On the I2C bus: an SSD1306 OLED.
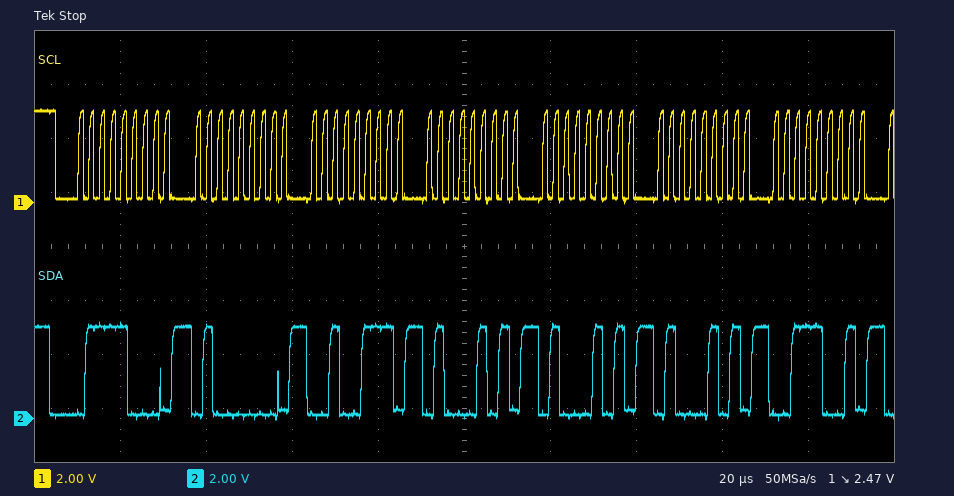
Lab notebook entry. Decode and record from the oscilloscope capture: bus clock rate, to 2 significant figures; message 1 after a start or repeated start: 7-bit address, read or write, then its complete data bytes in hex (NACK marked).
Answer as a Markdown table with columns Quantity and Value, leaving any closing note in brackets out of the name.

| Quantity | Value |
|---|---|
| bus clock rate, to 2 significant figures | 400 kHz |
| message 1 after a start or repeated start: 7-bit address, read or write, then its complete data bytes in hex | 0x3C write: 40 27 45 45 45 39 |
